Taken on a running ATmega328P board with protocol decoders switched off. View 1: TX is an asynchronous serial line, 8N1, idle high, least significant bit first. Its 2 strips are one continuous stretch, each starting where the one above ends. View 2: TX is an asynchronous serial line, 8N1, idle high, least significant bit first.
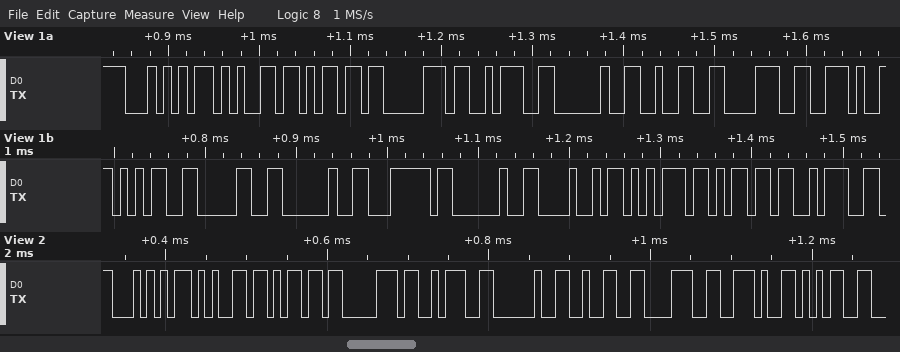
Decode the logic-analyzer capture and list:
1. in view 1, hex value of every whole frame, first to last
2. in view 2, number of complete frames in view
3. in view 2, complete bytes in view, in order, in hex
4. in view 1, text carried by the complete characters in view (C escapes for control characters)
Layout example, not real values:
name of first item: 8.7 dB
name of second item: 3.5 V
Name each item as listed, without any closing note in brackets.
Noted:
in view 1, hex value of every whole frame, first to last: 54 65 6D 70 3A 20 32 38 2E 35 30 20 7C 20 48 75 6D 3A
in view 2, number of complete frames in view: 10
in view 2, complete bytes in view, in order, in hex: 54 65 6D 70 3A 20 32 38 2E 35
in view 1, text carried by the complete characters in view: "Temp: 28.50 | Hum:"
